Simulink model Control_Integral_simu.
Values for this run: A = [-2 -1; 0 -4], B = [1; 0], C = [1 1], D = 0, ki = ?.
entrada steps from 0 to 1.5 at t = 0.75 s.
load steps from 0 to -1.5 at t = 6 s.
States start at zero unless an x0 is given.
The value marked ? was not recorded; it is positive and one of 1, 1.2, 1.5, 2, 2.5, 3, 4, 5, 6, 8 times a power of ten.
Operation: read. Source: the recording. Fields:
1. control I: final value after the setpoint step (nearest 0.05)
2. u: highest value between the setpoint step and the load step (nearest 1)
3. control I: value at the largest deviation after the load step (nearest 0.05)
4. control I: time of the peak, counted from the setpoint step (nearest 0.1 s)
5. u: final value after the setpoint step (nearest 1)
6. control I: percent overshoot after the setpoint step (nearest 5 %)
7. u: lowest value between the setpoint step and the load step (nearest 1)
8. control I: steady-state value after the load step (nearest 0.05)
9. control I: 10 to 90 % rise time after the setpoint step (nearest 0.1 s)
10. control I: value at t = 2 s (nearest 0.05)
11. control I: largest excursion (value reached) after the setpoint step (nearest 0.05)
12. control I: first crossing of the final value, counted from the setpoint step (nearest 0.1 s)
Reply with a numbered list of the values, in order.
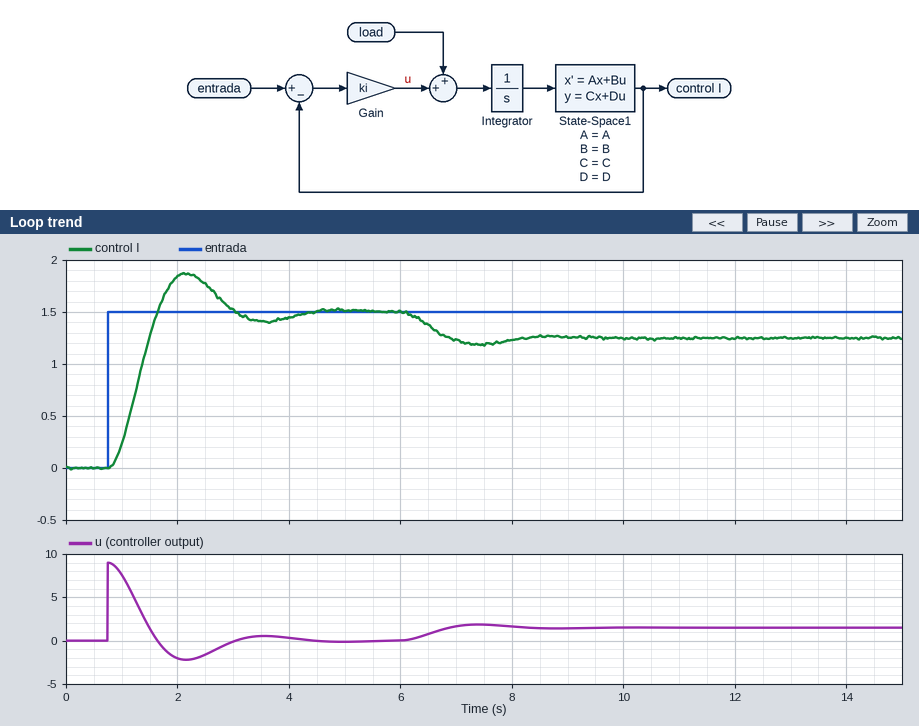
1. 1.50
2. 9
3. 1.20
4. 1.4 s
5. 0
6. 25 %
7. -2
8. 1.25
9. 0.6 s
10. 1.85
11. 1.85
12. 0.9 s
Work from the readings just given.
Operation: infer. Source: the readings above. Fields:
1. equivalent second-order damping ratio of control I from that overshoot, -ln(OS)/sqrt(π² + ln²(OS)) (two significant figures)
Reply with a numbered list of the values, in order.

1. 0.40
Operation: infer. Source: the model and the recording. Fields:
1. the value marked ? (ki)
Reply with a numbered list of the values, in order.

1. 6
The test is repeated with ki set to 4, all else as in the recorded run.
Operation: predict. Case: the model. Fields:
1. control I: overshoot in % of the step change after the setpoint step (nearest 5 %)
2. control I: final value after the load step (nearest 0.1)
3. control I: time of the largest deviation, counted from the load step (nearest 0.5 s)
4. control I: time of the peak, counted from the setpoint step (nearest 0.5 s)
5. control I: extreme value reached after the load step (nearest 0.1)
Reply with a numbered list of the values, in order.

1. 15 %
2. 1.1
3. 2.0 s
4. 2.0 s
5. 1.1
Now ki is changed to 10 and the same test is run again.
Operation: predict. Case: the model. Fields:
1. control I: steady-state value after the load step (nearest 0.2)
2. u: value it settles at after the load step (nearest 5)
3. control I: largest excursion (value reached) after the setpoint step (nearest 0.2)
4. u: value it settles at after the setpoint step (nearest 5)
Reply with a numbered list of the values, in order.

1. 1.4
2. 0
3. 2.0
4. 0
